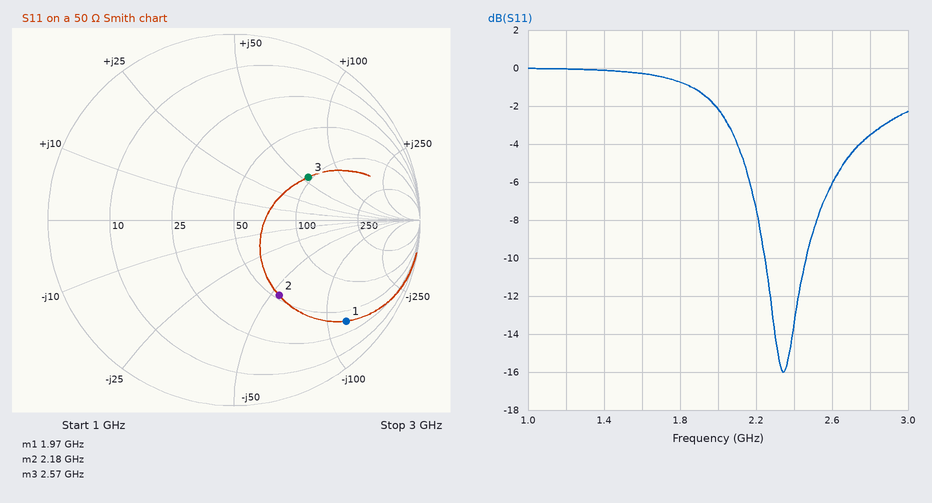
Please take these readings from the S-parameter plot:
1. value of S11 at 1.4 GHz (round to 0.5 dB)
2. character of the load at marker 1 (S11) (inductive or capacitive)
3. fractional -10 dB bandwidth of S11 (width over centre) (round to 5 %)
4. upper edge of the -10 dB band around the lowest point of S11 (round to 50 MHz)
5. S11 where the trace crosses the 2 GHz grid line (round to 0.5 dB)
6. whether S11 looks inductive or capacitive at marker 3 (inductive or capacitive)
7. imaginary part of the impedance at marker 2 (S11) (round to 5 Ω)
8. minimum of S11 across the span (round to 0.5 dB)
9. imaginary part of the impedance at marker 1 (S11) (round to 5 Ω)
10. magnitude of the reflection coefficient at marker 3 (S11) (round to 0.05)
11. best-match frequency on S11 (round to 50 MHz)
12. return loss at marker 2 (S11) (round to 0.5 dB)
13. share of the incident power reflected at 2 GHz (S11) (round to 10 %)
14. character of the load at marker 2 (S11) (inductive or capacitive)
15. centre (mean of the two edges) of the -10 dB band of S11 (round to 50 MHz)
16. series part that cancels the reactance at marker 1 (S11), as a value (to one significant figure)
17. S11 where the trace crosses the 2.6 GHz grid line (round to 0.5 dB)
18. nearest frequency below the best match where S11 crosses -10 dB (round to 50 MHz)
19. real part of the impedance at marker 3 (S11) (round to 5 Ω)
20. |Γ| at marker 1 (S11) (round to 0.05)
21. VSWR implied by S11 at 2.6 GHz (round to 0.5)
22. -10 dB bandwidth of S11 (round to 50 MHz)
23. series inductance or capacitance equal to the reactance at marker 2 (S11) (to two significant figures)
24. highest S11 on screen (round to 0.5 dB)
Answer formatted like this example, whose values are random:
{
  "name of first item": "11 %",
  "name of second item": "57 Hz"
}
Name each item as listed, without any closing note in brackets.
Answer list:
{
  "value of S11 at 1.4 GHz": "0.0 dB",
  "character of the load at marker 1 (S11)": "capacitive",
  "fractional -10 dB bandwidth of S11 (width over centre)": "10 %",
  "upper edge of the -10 dB band around the lowest point of S11": "2.45 GHz",
  "S11 where the trace crosses the 2 GHz grid line": "-2.0 dB",
  "whether S11 looks inductive or capacitive at marker 3": "inductive",
  "imaginary part of the impedance at marker 2 (S11)": "-55 Ω",
  "minimum of S11 across the span": "-16.0 dB",
  "imaginary part of the impedance at marker 1 (S11)": "-120 Ω",
  "magnitude of the reflection coefficient at marker 3 (S11)": "0.45",
  "best-match frequency on S11": "2.35 GHz",
  "return loss at marker 2 (S11)": "6.5 dB",
  "share of the incident power reflected at 2 GHz (S11)": "60 %",
  "character of the load at marker 2 (S11)": "capacitive",
  "centre (mean of the two edges) of the -10 dB band of S11": "2.35 GHz",
  "series part that cancels the reactance at marker 1 (S11), as a value": "10 nH",
  "S11 where the trace crosses the 2.6 GHz grid line": "-6.0 dB",
  "nearest frequency below the best match where S11 crosses -10 dB": "2.25 GHz",
  "real part of the impedance at marker 3 (S11)": "95 Ω",
  "|Γ| at marker 1 (S11)": "0.80",
  "VSWR implied by S11 at 2.6 GHz": "3.0",
  "-10 dB bandwidth of S11": "200 MHz",
  "series inductance or capacitance equal to the reactance at marker 2 (S11)": "1.3 pF",
  "highest S11 on screen": "0.0 dB"
}
